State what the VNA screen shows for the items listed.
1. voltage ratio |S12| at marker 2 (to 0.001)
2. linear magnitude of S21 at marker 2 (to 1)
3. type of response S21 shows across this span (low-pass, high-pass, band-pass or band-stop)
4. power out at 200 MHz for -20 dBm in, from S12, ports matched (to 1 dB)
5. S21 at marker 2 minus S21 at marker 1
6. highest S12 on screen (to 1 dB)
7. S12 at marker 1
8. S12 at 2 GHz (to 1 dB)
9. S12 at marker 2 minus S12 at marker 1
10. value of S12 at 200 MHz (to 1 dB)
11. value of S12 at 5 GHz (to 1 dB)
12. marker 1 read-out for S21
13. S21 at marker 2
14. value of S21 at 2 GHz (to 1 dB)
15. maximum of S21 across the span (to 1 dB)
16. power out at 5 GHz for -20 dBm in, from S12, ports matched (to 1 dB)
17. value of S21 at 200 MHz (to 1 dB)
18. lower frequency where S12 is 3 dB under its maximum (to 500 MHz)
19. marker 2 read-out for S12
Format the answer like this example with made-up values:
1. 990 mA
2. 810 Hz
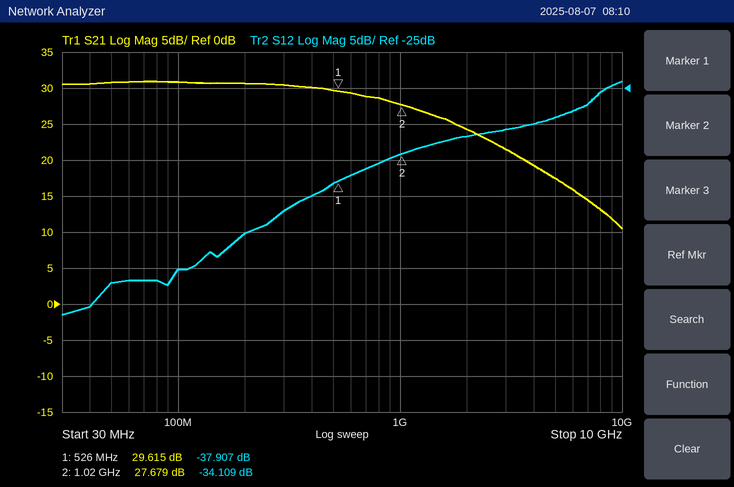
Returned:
1. 0.020
2. 24
3. low-pass
4. -65 dBm
5. -1.936 dB
6. -24 dB
7. -37.907 dB
8. -32 dB
9. 3.798 dB
10. -45 dB
11. -29 dB
12. 29.615 dB
13. 27.679 dB
14. 24 dB
15. 31 dB
16. -49 dBm
17. 31 dB
18. 7.0 GHz
19. -34.109 dB
